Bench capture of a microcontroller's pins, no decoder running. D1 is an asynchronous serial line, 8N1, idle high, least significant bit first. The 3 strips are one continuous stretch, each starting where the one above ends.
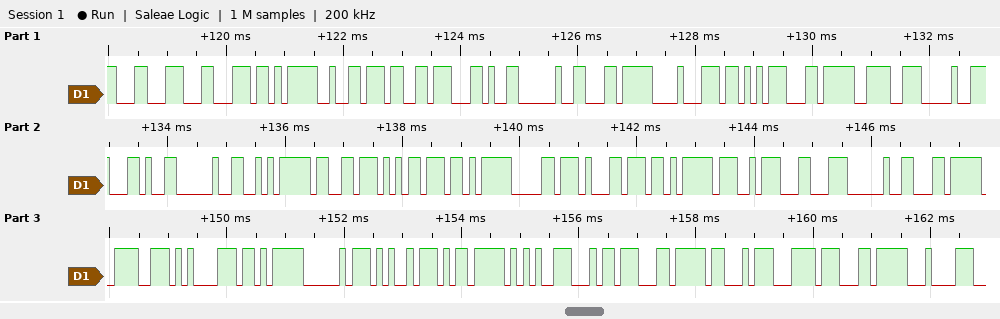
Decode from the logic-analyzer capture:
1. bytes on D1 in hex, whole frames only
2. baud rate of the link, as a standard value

8C 8C EB B2 B3 2C 20 EC 88 AB EC 9E 90 2C 20 EA B3 B5 EB B0 B1 EB A7 8C 20 EC 9E 85 EB A0 A5 ED 95 B4 EC A3 BC EC 84
9600 baud
